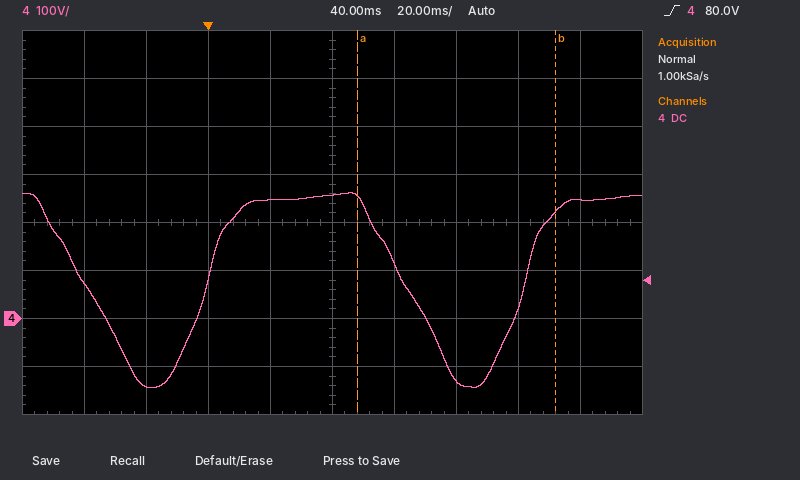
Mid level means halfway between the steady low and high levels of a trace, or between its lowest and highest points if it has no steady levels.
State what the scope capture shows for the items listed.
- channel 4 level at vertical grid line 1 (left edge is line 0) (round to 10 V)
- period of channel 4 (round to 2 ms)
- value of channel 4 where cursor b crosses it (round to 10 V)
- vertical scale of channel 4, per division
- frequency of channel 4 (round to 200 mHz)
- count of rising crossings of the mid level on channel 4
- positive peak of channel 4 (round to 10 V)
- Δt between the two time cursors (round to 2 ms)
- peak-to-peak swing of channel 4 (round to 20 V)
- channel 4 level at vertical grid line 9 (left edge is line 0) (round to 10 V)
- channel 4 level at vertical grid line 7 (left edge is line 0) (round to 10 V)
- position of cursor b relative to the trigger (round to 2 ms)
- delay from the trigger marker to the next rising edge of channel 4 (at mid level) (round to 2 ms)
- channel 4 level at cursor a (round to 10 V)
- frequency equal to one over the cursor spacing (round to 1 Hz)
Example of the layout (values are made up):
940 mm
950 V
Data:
70 V
102 ms
220 V
100 V
9.8 Hz
2
260 V
64 ms
400 V
250 V
-130 V
+112 ms
102 ms
250 V
16 Hz
